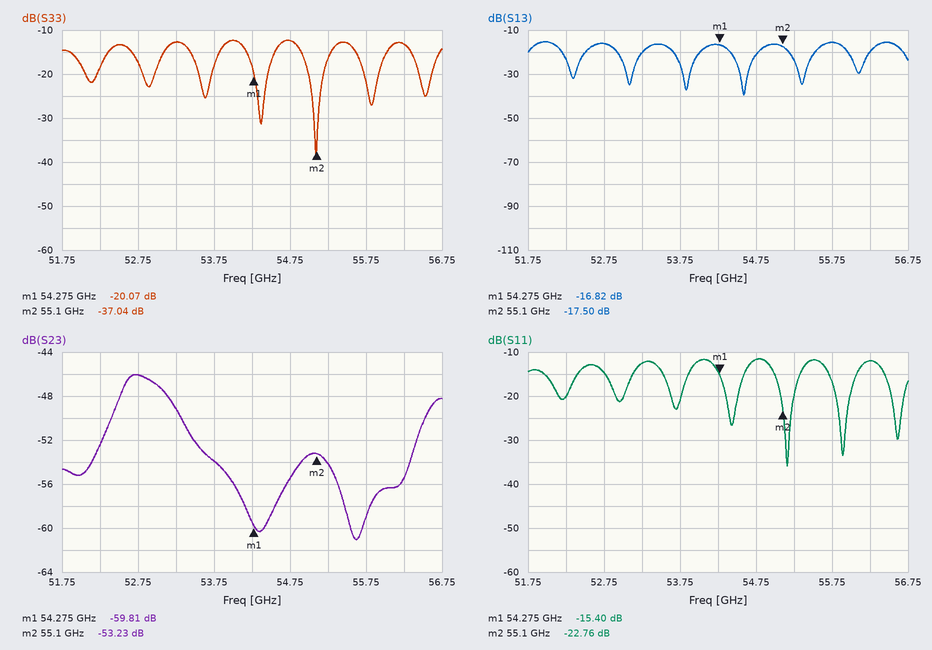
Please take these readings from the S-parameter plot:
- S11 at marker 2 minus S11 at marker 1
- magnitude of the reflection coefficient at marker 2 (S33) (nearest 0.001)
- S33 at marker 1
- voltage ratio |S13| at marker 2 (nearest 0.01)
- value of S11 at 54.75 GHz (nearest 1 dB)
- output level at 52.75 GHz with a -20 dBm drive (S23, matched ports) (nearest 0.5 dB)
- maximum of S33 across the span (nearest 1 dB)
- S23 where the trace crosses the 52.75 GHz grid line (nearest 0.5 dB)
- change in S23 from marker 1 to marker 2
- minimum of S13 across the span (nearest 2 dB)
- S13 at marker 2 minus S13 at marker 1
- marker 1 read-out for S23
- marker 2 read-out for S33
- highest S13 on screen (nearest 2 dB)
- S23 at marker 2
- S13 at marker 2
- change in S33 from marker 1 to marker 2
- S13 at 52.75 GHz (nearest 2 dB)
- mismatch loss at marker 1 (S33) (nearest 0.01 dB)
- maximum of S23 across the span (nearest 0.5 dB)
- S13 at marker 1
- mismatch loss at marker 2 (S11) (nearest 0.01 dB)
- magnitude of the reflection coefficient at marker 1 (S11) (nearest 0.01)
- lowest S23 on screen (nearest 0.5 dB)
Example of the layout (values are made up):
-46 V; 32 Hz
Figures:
-7.36 dB; 0.014; -20.07 dB; 0.13; -12 dB; -66.0 dBm; -12 dB; -46.0 dB; 6.58 dB; -40 dB; -0.68 dB; -59.81 dB; -37.04 dB; -16 dB; -53.23 dB; -17.50 dB; -16.97 dB; -16 dB; 0.04 dB; -46.0 dB; -16.82 dB; 0.02 dB; 0.17; -61.0 dB
